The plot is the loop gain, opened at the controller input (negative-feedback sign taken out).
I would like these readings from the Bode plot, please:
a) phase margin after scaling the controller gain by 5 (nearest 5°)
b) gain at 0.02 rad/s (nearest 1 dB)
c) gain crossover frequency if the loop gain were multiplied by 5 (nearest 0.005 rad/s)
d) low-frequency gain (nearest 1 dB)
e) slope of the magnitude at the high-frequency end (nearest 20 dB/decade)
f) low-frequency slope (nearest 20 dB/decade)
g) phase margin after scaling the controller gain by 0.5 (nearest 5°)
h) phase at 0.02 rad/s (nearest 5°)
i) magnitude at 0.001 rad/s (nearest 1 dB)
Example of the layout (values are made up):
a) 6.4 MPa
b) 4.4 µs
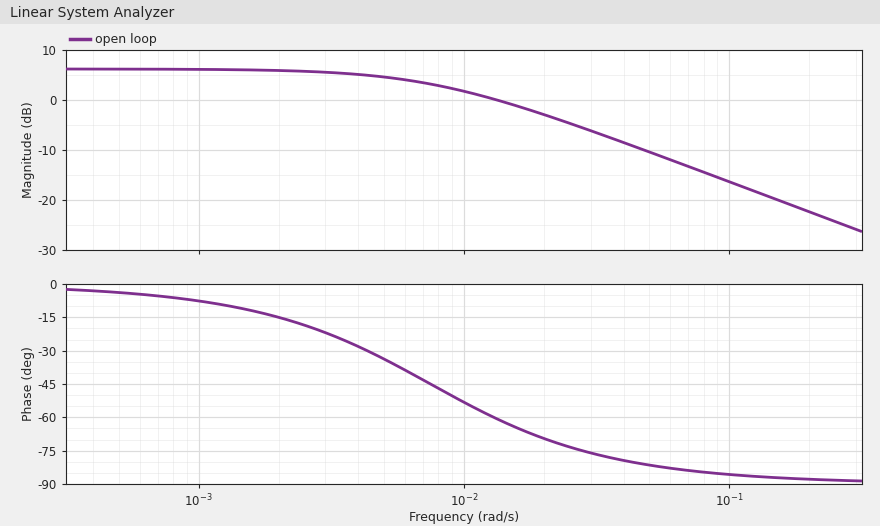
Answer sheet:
a) 95°
b) -3 dB
c) 0.075 rad/s
d) 6 dB
e) -20 dB/decade
f) 0 dB/decade
g) 170°
h) -70°
i) 6 dB
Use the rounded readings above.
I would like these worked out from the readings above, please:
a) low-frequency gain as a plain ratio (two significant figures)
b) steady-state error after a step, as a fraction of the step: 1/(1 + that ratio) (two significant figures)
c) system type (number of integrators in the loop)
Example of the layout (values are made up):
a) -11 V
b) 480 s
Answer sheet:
a) 2.0
b) 0.33
c) 0
